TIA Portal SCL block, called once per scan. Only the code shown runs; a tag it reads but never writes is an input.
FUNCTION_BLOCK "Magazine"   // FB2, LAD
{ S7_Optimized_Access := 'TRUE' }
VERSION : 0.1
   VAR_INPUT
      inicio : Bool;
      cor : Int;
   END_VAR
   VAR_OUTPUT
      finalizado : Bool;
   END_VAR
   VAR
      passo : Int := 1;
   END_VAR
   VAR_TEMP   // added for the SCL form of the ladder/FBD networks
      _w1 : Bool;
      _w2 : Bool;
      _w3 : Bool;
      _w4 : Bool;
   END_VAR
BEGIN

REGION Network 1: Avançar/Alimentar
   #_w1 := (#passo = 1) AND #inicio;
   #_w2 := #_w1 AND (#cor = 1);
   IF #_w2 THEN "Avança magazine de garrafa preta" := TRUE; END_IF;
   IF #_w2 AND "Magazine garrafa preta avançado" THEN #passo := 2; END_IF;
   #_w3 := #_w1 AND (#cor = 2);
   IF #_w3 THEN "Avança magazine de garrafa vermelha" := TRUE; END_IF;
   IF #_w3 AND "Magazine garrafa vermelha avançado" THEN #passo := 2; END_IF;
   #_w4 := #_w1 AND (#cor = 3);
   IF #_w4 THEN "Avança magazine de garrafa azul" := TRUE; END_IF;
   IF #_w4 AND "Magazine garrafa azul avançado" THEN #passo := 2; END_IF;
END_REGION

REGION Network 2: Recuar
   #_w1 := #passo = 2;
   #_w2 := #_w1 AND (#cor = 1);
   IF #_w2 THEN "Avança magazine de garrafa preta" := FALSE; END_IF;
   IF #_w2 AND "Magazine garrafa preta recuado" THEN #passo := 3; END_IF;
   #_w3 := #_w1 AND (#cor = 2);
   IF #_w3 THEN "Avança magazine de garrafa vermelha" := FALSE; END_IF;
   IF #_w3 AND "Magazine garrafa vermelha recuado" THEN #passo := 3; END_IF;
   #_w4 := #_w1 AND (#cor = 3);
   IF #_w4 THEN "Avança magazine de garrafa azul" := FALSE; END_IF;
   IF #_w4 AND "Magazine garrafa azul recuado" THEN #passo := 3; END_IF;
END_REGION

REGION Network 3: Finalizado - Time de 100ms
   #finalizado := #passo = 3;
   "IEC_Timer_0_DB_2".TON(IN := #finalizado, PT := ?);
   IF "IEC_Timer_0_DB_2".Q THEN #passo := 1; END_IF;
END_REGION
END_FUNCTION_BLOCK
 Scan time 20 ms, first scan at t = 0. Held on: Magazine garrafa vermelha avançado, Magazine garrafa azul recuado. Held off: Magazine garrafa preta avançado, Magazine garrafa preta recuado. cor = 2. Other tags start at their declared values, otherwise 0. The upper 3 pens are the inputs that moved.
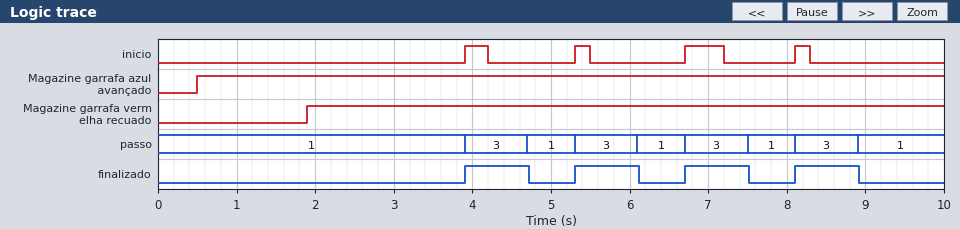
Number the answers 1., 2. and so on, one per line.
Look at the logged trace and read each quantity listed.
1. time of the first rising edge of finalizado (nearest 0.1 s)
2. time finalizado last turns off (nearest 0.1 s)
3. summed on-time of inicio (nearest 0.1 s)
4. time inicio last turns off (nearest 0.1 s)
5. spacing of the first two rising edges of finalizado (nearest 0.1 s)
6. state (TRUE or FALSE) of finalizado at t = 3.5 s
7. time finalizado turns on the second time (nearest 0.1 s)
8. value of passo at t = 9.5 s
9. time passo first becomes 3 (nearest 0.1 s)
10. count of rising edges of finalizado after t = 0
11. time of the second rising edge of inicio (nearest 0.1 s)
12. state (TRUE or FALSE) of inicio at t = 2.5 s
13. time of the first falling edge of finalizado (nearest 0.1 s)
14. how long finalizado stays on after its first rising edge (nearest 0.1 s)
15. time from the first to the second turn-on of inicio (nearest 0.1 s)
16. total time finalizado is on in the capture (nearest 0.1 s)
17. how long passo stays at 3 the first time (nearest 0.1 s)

1. 3.9 s
2. 8.9 s
3. 1.2 s
4. 8.3 s
5. 1.4 s
6. FALSE
7. 5.3 s
8. 1
9. 3.9 s
10. 4
11. 5.3 s
12. FALSE
13. 4.7 s
14. 0.8 s
15. 1.4 s
16. 3.3 s
17. 0.8 s
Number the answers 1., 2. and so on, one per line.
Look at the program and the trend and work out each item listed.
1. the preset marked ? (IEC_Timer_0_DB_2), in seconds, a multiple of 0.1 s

1. 0.8 s
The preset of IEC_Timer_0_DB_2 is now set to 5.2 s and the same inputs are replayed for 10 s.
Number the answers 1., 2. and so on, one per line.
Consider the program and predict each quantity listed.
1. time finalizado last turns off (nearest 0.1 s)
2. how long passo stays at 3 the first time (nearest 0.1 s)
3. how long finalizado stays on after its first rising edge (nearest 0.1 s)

1. 9.1 s
2. 5.2 s
3. 5.2 s
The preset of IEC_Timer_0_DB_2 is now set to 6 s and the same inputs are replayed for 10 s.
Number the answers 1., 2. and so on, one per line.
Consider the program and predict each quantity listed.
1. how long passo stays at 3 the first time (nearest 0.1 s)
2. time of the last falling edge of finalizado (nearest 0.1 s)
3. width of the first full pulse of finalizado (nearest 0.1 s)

1. 6.0 s
2. 9.9 s
3. 6.0 s
